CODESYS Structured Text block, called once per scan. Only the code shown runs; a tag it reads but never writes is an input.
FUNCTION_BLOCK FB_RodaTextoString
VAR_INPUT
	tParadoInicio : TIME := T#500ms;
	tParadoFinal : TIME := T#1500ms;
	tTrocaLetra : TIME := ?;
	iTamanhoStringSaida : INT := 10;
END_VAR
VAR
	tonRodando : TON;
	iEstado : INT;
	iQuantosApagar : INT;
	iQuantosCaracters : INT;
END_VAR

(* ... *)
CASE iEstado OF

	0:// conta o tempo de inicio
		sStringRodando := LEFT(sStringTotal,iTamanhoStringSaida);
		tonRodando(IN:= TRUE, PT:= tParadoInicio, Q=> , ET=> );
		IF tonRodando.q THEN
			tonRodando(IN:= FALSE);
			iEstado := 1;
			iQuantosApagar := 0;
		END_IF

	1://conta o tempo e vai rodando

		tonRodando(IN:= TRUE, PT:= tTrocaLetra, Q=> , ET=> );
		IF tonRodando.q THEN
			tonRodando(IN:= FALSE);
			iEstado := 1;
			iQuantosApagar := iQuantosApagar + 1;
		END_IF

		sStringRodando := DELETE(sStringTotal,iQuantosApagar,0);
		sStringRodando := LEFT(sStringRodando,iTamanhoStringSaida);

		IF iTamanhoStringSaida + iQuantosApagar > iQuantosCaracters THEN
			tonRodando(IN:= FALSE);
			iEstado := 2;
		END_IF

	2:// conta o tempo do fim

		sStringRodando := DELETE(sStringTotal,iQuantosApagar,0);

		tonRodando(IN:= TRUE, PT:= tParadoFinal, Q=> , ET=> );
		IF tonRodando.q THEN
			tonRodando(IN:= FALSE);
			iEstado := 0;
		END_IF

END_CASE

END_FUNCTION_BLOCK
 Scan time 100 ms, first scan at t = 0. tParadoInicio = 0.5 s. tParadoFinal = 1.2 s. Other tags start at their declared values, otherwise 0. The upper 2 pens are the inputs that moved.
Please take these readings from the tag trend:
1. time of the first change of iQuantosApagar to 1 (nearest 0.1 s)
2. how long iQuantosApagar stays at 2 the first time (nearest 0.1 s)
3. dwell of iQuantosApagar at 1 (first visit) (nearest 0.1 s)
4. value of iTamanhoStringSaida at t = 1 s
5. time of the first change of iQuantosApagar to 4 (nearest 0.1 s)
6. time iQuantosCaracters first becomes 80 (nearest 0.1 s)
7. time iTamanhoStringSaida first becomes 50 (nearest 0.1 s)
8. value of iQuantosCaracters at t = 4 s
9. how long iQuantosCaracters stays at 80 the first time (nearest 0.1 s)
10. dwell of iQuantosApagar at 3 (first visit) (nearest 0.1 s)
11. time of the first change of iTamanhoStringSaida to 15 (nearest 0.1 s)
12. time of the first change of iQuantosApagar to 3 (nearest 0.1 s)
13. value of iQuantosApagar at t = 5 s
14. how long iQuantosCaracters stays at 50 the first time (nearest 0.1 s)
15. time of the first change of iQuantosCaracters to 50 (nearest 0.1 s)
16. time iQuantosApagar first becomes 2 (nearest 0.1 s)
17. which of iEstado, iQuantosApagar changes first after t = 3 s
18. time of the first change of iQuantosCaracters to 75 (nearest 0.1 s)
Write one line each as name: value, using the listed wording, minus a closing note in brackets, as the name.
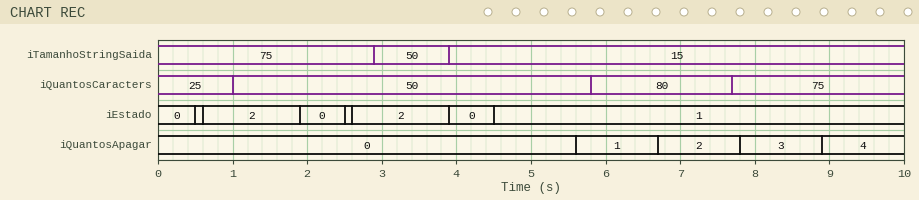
time of the first change of iQuantosApagar to 1: 5.6 s
how long iQuantosApagar stays at 2 the first time: 1.1 s
dwell of iQuantosApagar at 1 (first visit): 1.1 s
value of iTamanhoStringSaida at t = 1 s: 75
time of the first change of iQuantosApagar to 4: 8.9 s
time iQuantosCaracters first becomes 80: 5.8 s
time iTamanhoStringSaida first becomes 50: 2.9 s
value of iQuantosCaracters at t = 4 s: 50
how long iQuantosCaracters stays at 80 the first time: 1.9 s
dwell of iQuantosApagar at 3 (first visit): 1.1 s
time of the first change of iTamanhoStringSaida to 15: 3.9 s
time of the first change of iQuantosApagar to 3: 7.8 s
value of iQuantosApagar at t = 5 s: 0
how long iQuantosCaracters stays at 50 the first time: 4.8 s
time of the first change of iQuantosCaracters to 50: 1.0 s
time iQuantosApagar first becomes 2: 6.7 s
which of iEstado, iQuantosApagar changes first after t = 3 s: iEstado
time of the first change of iQuantosCaracters to 75: 7.7 s
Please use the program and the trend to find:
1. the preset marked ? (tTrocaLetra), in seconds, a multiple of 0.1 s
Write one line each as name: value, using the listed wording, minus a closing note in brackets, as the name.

the preset marked ? (tTrocaLetra), in seconds, a multiple of 0.1 s: 1.0 s
